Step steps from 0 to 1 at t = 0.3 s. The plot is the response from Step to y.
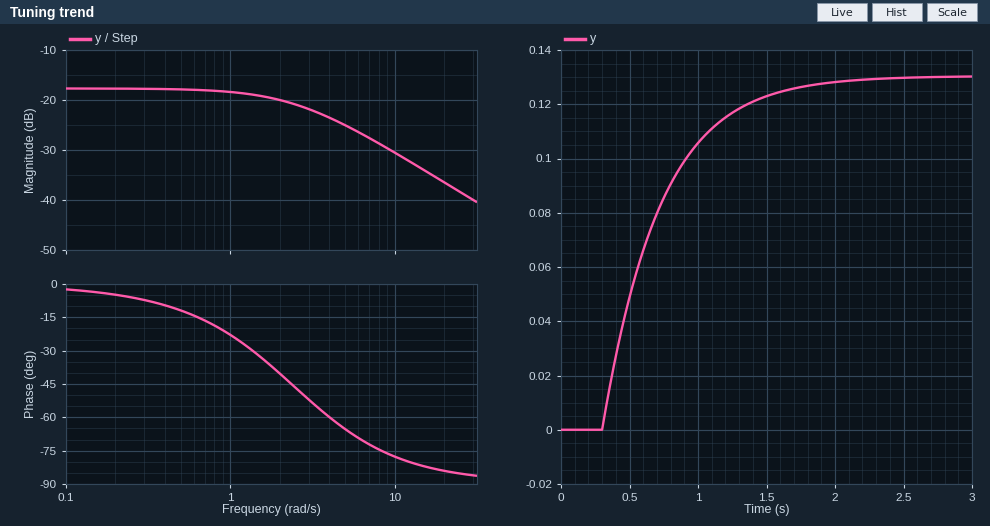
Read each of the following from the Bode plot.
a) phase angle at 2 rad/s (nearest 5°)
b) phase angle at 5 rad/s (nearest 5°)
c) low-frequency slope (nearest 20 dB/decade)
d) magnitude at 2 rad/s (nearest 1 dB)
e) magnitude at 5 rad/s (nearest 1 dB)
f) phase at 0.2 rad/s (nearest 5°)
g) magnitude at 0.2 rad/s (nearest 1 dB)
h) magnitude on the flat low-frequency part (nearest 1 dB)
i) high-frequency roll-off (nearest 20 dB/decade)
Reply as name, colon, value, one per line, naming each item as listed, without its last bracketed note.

phase angle at 2 rad/s: -40°
phase angle at 5 rad/s: -65°
low-frequency slope: 0 dB/decade
magnitude at 2 rad/s: -20 dB
magnitude at 5 rad/s: -25 dB
phase at 0.2 rad/s: -5°
magnitude at 0.2 rad/s: -18 dB
magnitude on the flat low-frequency part: -18 dB
high-frequency roll-off: -20 dB/decade
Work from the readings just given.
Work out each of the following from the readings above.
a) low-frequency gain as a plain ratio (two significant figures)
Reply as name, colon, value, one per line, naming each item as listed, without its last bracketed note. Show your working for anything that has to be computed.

low-frequency gain as a plain ratio: 10^(-18 / 20) = 0.13
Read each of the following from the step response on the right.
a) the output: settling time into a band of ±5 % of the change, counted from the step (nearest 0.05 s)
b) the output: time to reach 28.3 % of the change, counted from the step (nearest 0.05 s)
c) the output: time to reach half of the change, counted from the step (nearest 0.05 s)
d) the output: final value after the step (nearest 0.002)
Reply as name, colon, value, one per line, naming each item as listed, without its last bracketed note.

the output: settling time into a band of ±5 % of the change, counted from the step: 1.25 s
the output: time to reach 28.3 % of the change, counted from the step: 0.15 s
the output: time to reach half of the change, counted from the step: 0.30 s
the output: final value after the step: 0.130
